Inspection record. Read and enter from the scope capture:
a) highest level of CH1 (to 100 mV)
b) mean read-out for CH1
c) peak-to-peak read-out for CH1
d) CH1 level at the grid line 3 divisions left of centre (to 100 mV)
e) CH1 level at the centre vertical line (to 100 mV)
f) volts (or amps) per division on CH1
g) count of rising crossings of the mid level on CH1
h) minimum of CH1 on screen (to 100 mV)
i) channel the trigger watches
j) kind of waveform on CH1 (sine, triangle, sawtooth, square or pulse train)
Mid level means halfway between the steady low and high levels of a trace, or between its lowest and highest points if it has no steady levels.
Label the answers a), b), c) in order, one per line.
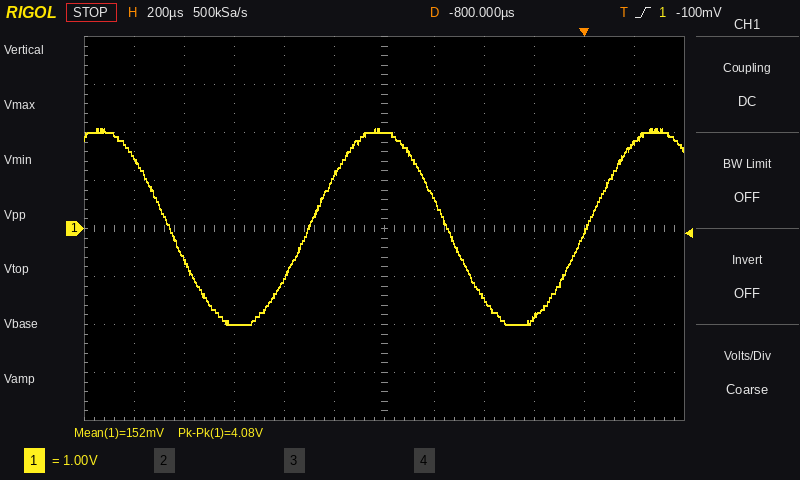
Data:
a) 2.1 V
b) 152 mV
c) 4.08 V
d) -2.0 V
e) 2.0 V
f) 1 V
g) 2
h) -2.0 V
i) CH1
j) sine
